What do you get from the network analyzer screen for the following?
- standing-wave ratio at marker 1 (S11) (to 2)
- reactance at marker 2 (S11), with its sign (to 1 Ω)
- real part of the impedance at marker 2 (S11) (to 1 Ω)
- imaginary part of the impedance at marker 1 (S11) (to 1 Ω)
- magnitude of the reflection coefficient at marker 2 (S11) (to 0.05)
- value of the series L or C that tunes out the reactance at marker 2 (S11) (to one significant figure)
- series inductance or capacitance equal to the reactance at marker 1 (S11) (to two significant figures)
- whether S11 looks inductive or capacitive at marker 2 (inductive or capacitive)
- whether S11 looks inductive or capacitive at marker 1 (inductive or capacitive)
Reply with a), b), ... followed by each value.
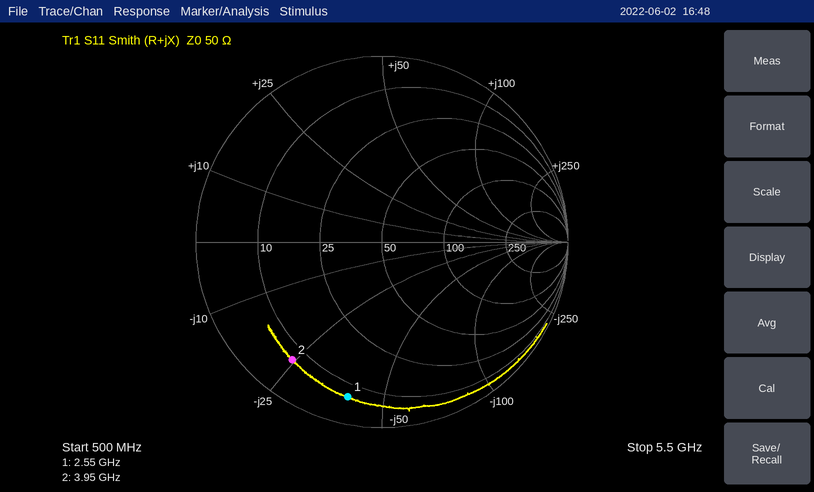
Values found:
a) 12
b) -24 Ω
c) 7 Ω
d) -40 Ω
e) 0.80
f) 1.0 nH
g) 1.6 pF
h) capacitive
i) capacitive
